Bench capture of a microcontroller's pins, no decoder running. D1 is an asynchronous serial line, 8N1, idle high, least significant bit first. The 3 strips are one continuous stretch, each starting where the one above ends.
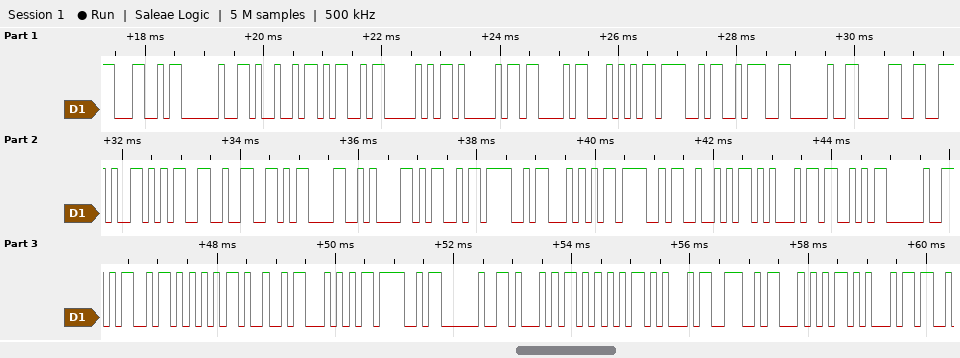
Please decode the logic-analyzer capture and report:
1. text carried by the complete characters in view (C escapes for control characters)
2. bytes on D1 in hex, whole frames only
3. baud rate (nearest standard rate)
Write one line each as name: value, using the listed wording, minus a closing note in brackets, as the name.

text carried by the complete characters in view: "L IMPACTO: 0.52\r\nMOTORES MUITO QUENTE"
bytes on D1 in hex, whole frames only: 4C 20 49 4D 50 41 43 54 4F 3A 20 30 2E 35 32 0D 0A 4D 4F 54 4F 52 45 53 20 4D 55 49 54 4F 20 51 55 45 4E 54 45
baud rate: 9600 baud
